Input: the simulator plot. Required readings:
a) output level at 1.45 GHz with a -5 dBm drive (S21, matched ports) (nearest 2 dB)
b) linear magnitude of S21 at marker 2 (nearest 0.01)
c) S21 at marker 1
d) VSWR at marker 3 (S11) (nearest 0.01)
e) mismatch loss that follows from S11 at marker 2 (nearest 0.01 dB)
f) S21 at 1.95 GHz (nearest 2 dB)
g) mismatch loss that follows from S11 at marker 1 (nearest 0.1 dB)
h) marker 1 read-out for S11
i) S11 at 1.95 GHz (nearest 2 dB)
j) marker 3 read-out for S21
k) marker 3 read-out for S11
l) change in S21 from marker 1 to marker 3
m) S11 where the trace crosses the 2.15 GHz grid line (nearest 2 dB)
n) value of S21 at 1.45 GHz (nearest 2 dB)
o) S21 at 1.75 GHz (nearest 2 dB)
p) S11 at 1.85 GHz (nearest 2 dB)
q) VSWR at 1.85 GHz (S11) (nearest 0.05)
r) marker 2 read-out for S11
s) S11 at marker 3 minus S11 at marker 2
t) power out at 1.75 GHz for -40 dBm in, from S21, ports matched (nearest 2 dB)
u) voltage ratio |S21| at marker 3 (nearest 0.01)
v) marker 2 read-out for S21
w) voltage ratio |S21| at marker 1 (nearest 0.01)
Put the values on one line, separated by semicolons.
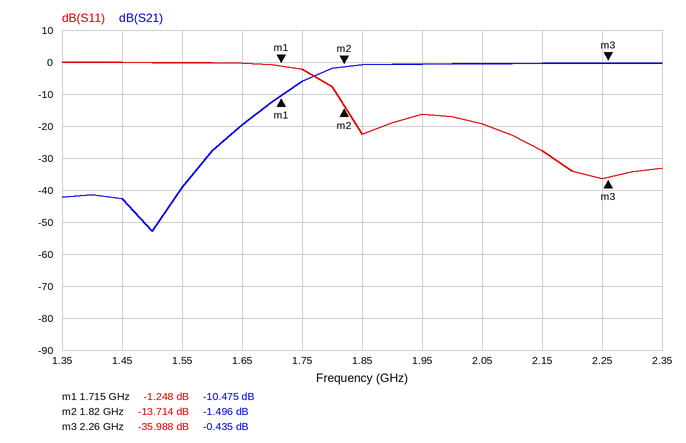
-48 dBm; 0.84; -10.475 dB; 1.03; 0.19 dB; 0 dB; 6.0 dB; -1.248 dB; -16 dB; -0.435 dB; -35.988 dB; 10.040 dB; -28 dB; -42 dB; -6 dB; -22 dB; 1.15; -13.714 dB; -22.274 dB; -46 dBm; 0.95; -1.496 dB; 0.30
